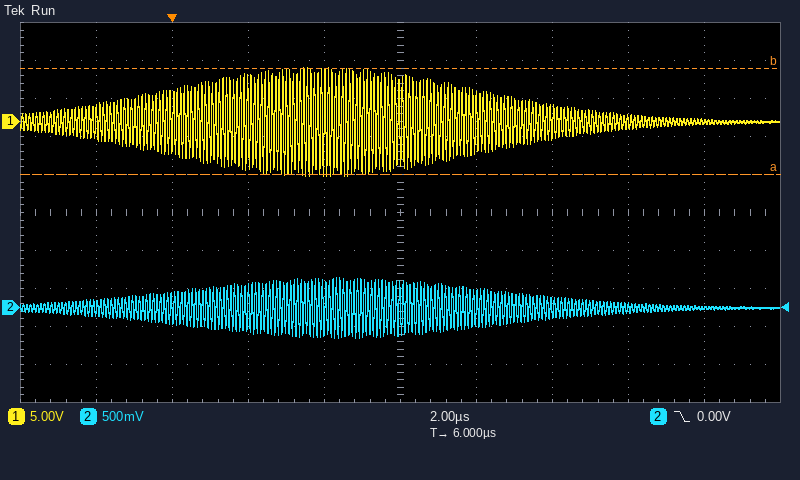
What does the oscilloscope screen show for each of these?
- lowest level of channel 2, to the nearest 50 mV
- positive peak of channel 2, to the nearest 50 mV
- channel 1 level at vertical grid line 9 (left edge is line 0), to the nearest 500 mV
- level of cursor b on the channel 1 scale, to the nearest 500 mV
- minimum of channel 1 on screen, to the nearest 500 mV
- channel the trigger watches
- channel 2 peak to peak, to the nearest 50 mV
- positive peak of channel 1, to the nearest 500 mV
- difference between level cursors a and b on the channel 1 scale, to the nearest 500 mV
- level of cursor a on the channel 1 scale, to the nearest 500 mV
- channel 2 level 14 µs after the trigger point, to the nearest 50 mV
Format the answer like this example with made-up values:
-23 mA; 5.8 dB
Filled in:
-400 mV; 400 mV; 0.0 V; 7.0 V; -7.0 V; channel 2; 800 mV; 7.0 V; 14.0 V; -7.0 V; 0 mV
